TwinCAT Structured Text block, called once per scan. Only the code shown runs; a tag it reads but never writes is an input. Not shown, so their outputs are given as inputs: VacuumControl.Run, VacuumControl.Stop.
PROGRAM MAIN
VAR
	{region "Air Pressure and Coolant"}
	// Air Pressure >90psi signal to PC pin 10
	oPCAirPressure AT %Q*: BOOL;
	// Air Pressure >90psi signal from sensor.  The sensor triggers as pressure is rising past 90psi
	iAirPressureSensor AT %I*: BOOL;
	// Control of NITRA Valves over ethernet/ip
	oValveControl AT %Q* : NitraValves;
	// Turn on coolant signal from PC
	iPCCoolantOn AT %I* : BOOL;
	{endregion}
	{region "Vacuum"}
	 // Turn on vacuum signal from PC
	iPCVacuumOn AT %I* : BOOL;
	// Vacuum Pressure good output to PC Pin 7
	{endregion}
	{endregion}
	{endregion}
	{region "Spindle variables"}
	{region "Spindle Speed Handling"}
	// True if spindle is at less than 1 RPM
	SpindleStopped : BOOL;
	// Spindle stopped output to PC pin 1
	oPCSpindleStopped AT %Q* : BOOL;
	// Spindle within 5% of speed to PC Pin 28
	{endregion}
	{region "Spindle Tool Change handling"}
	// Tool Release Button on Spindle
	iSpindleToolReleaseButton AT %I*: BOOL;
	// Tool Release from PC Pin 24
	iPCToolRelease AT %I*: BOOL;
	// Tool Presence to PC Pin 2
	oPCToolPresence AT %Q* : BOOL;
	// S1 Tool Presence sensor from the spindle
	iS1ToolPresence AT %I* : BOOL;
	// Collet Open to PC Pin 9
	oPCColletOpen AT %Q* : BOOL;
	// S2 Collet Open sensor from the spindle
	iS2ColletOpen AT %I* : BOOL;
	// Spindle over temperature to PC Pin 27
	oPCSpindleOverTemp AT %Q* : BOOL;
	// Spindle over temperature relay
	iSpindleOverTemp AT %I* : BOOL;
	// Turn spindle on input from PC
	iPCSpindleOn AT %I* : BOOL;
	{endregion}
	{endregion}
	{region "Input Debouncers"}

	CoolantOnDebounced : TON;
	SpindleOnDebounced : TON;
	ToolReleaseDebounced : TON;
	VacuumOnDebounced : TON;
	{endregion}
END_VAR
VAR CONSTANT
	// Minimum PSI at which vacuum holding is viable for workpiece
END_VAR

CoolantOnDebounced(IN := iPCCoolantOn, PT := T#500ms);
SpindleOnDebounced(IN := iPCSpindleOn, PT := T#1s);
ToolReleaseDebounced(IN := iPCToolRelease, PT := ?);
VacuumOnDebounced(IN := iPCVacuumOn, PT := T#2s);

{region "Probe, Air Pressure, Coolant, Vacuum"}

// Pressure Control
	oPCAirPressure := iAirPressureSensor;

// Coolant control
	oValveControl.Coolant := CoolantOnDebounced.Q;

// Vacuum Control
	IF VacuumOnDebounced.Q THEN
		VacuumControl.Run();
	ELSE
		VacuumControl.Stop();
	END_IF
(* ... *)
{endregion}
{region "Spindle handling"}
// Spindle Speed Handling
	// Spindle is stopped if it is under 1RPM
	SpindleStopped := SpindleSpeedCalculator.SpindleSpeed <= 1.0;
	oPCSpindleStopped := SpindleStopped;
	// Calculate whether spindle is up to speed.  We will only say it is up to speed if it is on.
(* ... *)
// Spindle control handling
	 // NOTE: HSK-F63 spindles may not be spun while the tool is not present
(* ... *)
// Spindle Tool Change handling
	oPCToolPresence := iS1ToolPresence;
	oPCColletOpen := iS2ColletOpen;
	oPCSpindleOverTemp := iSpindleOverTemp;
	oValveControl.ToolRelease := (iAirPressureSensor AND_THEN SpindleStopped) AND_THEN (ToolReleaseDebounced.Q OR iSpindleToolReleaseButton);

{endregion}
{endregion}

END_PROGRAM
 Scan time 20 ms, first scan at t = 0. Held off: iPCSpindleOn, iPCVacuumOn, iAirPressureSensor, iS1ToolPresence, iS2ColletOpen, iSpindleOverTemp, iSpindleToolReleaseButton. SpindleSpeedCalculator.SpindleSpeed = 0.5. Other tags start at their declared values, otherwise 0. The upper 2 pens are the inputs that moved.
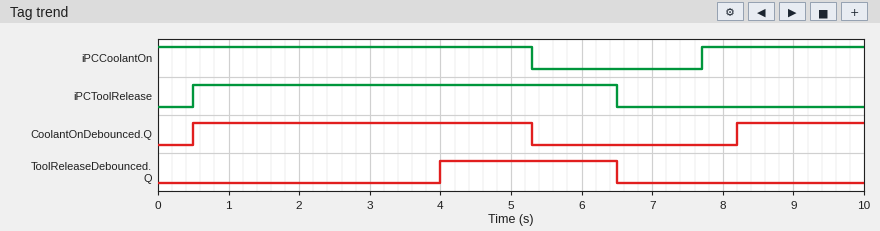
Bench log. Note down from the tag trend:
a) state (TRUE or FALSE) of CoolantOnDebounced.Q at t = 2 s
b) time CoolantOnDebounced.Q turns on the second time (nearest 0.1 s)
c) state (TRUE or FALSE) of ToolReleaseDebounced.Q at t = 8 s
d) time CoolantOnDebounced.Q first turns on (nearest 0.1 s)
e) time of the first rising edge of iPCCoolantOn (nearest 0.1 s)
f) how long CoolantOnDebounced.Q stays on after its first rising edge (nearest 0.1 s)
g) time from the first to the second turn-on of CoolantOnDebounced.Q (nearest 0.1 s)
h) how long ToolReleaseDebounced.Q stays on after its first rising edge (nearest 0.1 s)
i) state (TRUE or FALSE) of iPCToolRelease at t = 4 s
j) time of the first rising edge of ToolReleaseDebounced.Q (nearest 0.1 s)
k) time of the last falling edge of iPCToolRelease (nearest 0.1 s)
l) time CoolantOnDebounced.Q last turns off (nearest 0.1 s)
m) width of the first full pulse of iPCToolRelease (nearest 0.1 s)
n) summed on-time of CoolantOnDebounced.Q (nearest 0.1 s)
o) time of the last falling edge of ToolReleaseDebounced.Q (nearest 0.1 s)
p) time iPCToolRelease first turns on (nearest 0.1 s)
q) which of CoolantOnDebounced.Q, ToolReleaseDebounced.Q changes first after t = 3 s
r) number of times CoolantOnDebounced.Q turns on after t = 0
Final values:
TRUE
8.2 s
FALSE
0.5 s
7.7 s
4.8 s
7.7 s
2.5 s
TRUE
4.0 s
6.5 s
5.3 s
6.0 s
6.6 s
6.5 s
0.5 s
ToolReleaseDebounced.Q
2
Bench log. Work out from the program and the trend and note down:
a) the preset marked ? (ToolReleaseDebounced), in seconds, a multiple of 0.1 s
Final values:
3.5 s
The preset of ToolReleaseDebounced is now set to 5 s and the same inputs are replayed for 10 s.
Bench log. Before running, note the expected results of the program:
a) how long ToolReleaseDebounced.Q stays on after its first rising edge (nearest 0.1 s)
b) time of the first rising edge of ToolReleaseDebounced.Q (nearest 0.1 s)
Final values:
1.0 s
5.5 s
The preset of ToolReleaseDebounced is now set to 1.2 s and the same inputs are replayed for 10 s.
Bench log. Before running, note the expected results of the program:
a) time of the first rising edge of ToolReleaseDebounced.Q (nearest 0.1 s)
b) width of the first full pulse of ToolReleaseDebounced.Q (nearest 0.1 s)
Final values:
1.7 s
4.8 s
